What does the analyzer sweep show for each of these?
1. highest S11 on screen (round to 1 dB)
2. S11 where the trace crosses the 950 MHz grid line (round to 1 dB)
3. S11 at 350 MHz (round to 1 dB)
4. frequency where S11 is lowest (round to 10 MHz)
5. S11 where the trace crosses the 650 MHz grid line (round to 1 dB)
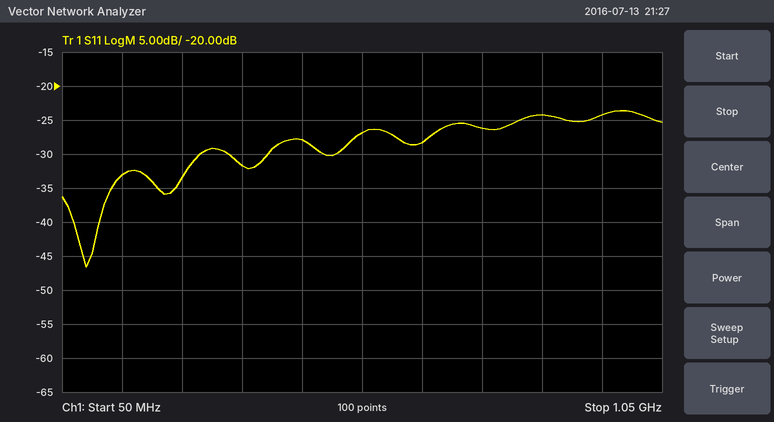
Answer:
-24 dB
-24 dB
-32 dB
90 MHz
-28 dB
